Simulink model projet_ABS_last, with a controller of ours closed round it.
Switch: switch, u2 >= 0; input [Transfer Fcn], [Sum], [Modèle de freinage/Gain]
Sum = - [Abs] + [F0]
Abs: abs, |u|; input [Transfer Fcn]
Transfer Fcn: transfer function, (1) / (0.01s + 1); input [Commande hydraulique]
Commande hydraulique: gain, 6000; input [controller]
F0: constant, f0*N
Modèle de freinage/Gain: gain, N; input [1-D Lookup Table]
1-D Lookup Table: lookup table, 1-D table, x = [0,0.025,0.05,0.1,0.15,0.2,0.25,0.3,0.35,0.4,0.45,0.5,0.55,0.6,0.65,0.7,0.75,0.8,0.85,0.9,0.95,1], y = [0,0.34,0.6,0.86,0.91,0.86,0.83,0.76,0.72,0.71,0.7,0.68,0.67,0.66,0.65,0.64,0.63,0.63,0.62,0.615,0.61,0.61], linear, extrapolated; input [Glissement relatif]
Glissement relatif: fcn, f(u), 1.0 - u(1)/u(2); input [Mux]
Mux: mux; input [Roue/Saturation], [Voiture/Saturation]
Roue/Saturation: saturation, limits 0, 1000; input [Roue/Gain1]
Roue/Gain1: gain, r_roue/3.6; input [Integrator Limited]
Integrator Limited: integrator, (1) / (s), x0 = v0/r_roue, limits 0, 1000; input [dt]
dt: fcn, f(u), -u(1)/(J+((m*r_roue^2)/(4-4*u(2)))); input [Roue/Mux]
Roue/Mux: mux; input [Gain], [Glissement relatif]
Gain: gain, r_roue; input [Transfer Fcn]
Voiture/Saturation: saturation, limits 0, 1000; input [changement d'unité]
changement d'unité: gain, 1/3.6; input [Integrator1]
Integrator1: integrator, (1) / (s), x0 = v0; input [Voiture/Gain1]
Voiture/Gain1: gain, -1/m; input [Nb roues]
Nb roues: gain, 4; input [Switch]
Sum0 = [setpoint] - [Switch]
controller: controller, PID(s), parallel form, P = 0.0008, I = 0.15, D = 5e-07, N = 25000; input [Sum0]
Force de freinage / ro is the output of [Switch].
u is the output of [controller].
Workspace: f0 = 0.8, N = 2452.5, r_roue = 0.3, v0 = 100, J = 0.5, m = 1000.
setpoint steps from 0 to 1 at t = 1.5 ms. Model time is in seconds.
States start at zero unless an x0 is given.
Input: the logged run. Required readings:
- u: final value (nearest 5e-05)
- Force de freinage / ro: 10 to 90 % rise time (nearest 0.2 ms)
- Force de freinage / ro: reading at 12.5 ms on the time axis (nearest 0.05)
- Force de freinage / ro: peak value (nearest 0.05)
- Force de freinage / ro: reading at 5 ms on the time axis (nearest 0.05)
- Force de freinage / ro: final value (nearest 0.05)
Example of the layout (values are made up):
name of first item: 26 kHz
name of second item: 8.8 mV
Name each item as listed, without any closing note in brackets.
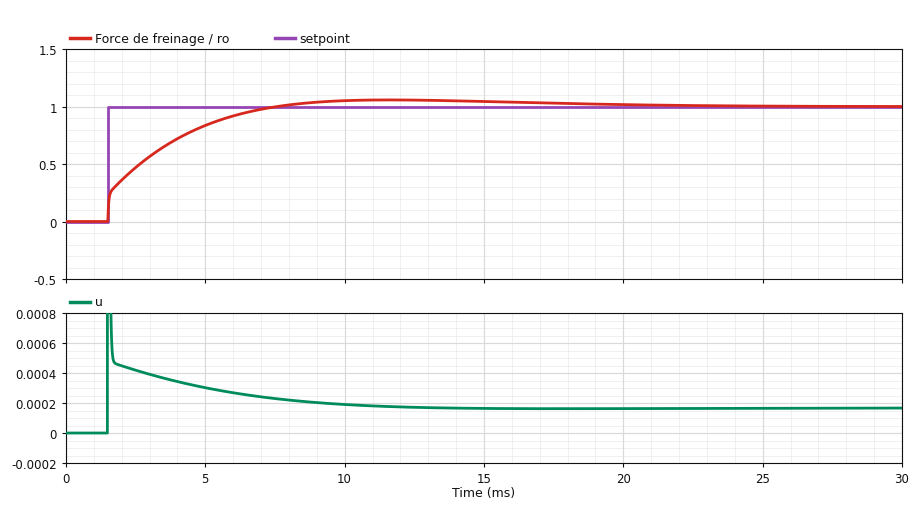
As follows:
u: final value: 0.00015
Force de freinage / ro: 10 to 90 % rise time: 4.2 ms
Force de freinage / ro: reading at 12.5 ms on the time axis: 1.05
Force de freinage / ro: peak value: 1.05
Force de freinage / ro: reading at 5 ms on the time axis: 0.85
Force de freinage / ro: final value: 1.00
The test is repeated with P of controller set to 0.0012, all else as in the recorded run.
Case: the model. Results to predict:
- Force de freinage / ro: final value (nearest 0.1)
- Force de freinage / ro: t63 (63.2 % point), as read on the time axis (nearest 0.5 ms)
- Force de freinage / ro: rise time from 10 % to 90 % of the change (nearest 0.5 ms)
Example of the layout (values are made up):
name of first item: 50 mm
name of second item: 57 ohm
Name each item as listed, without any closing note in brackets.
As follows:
Force de freinage / ro: final value: 1.0
Force de freinage / ro: t63 (63.2 % point), as read on the time axis: 3.0 ms
Force de freinage / ro: rise time from 10 % to 90 % of the change: 3.5 ms
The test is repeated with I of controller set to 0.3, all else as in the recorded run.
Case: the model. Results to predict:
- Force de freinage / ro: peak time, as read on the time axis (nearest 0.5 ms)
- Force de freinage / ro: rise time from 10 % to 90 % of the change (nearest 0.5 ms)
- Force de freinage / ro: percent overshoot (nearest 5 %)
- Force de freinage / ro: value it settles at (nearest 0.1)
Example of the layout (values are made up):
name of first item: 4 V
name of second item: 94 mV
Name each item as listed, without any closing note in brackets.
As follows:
Force de freinage / ro: peak time, as read on the time axis: 8.5 ms
Force de freinage / ro: rise time from 10 % to 90 % of the change: 3.0 ms
Force de freinage / ro: percent overshoot: 15 %
Force de freinage / ro: value it settles at: 1.0
